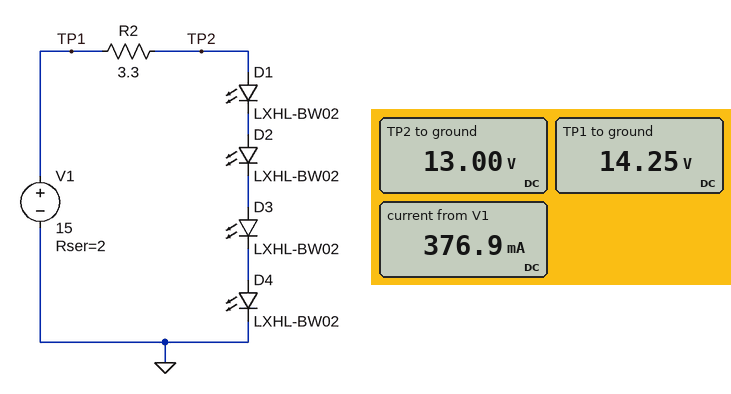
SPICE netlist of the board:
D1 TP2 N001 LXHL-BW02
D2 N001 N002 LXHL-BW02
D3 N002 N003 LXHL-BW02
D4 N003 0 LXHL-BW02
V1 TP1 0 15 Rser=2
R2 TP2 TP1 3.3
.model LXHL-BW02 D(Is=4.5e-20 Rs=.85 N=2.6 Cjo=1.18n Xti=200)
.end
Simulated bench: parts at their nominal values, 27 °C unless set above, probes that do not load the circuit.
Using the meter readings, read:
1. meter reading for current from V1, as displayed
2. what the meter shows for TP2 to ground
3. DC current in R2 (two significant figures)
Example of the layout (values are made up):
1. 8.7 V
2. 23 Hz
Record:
1. 376.9 mA
2. 13.00 V
3. 380 mA
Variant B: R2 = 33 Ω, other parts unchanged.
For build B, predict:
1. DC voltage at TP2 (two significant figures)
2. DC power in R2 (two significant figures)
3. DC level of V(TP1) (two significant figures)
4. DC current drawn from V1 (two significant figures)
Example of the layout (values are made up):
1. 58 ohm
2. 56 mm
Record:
1. 12 V
2. 300 mW
3. 15 V
4. 95 mA
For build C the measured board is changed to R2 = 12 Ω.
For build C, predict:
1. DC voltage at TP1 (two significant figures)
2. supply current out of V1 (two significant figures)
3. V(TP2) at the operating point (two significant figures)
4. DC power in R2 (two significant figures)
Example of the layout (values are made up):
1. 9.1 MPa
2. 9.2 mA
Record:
1. 15 V
2. 200 mA
3. 12 V
4. 470 mW
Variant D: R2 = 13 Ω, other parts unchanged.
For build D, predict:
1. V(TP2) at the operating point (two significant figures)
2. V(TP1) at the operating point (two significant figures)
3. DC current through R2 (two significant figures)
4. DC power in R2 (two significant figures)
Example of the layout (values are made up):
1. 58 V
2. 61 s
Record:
1. 12 V
2. 15 V
3. 190 mA
4. 460 mW
